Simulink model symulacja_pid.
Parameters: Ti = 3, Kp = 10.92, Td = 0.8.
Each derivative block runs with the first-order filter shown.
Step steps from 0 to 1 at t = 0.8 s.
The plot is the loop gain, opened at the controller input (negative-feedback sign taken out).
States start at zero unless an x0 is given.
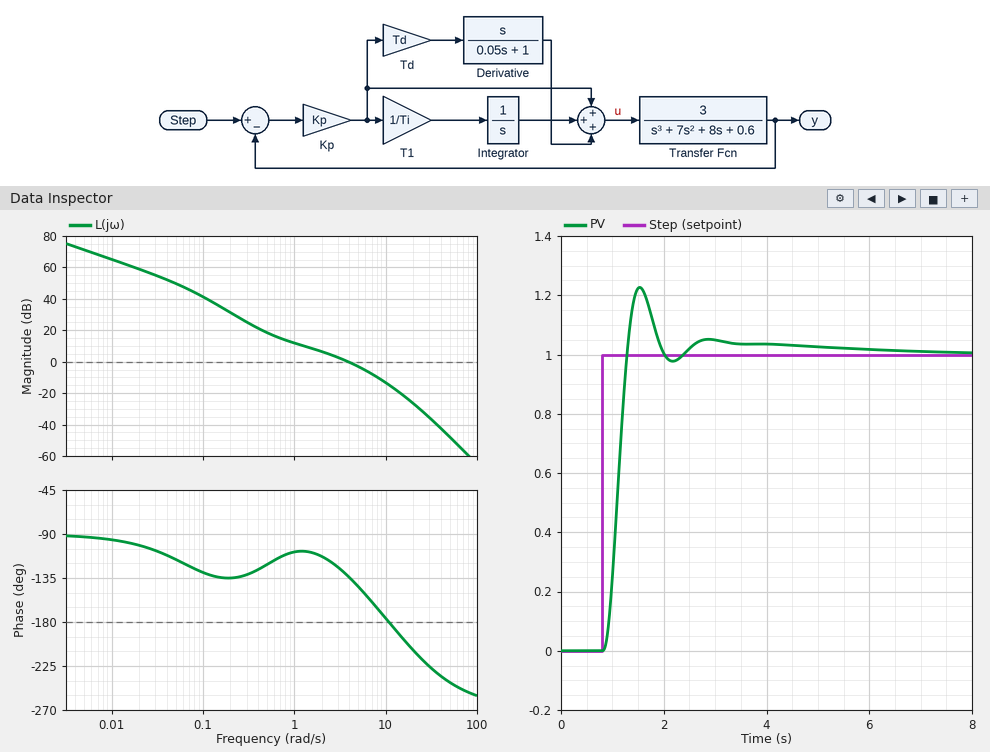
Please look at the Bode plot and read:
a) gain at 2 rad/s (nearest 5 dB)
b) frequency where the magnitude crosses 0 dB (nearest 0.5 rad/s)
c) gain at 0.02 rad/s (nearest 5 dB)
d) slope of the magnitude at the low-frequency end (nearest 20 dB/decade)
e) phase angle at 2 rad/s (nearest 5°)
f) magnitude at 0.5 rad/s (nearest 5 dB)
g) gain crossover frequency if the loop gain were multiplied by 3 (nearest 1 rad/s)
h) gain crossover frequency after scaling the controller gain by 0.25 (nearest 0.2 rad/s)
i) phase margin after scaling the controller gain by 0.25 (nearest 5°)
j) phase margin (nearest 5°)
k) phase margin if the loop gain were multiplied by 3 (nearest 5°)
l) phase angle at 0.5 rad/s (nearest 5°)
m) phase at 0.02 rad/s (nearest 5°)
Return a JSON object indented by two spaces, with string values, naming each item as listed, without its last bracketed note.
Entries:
{
  "gain at 2 rad/s": "5 dB",
  "frequency where the magnitude crosses 0 dB": "4.0 rad/s",
  "gain at 0.02 rad/s": "60 dB",
  "slope of the magnitude at the low-frequency end": "-20 dB/decade",
  "phase angle at 2 rad/s": "-115°",
  "magnitude at 0.5 rad/s": "20 dB",
  "gain crossover frequency if the loop gain were multiplied by 3": "8 rad/s",
  "gain crossover frequency after scaling the controller gain by 0.25": "1.0 rad/s",
  "phase margin after scaling the controller gain by 0.25": "70°",
  "phase margin": "45°",
  "phase margin if the loop gain were multiplied by 3": "15°",
  "phase angle at 0.5 rad/s": "-120°",
  "phase at 0.02 rad/s": "-100°"
}
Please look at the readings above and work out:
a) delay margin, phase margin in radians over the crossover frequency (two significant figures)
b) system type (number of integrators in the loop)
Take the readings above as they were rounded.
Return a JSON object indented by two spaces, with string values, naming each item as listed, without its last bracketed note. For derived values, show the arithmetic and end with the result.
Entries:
{
  "delay margin, phase margin in radians over the crossover frequency": "45 × π / 180 / 4 = 0.20 s",
  "system type": "1"
}
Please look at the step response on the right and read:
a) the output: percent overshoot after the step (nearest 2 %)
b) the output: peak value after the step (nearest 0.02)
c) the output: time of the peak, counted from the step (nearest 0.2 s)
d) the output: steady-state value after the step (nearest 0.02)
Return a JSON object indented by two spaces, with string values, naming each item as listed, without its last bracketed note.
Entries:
{
  "the output: percent overshoot after the step": "22 %",
  "the output: peak value after the step": "1.22",
  "the output: time of the peak, counted from the step": "0.8 s",
  "the output: steady-state value after the step": "1.00"
}
